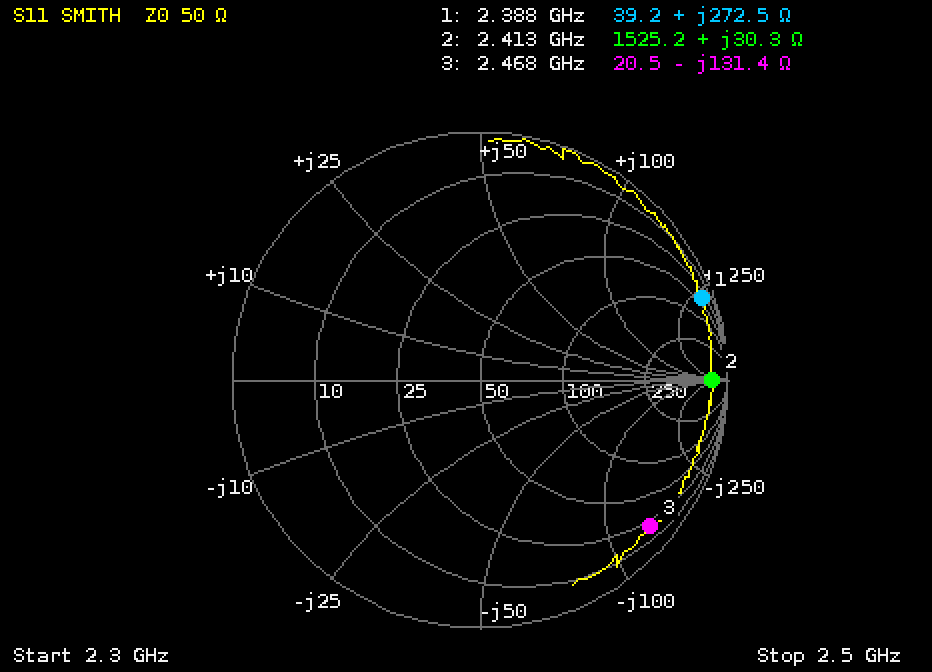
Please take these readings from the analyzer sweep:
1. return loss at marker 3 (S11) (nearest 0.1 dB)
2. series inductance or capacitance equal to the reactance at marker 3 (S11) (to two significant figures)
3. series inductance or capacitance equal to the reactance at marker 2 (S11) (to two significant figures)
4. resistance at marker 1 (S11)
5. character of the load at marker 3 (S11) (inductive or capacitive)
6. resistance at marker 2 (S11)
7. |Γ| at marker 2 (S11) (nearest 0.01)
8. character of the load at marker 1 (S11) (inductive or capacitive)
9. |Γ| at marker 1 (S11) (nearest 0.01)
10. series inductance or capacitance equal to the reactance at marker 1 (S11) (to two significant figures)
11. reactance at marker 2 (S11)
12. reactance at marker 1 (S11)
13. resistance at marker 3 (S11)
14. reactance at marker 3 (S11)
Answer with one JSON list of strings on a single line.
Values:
["0.9 dB", "490 fF", "2.0 nH", "39.2 Ω", "capacitive", "1525.2 Ω", "0.94", "inductive", "0.95", "18 nH", "+30.3 Ω", "+272.5 Ω", "20.5 Ω", "-131.4 Ω"]
